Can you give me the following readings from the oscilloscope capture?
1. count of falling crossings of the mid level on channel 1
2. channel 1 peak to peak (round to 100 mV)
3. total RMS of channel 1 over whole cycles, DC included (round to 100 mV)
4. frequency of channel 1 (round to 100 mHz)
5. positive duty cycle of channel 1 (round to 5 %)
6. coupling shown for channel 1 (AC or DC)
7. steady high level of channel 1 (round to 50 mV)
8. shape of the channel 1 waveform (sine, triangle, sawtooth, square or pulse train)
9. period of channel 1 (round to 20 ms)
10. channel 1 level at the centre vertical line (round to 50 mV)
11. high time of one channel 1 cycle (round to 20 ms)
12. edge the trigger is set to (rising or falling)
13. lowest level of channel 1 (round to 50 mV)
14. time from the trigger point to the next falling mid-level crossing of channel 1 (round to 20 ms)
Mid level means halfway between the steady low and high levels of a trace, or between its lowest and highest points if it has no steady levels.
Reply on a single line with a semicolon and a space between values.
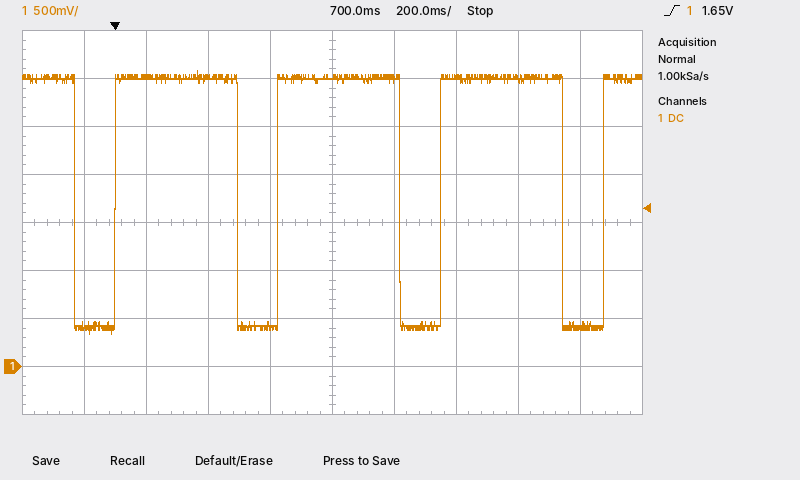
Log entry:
4; 2.70 V; 2.6 V; 1.9 Hz; 75 %; DC; 3.00 V; pulse train; 520 ms; 3.00 V; 400 ms; rising; 350 mV; 400 ms
